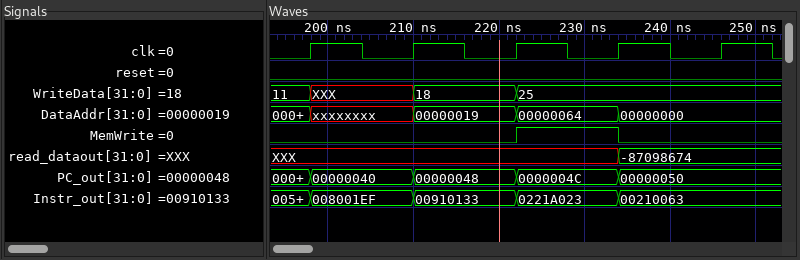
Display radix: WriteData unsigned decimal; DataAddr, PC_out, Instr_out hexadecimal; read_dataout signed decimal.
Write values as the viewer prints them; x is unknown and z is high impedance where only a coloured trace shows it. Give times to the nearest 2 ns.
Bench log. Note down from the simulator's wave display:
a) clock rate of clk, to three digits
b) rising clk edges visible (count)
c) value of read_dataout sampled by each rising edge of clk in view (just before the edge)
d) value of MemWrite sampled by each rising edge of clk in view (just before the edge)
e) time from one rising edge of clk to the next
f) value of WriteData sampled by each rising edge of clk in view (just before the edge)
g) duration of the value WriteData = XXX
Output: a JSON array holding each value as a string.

["83.3 MHz", "5", "XXX, XXX, XXX, XXX, -87098674", "0 0 0 1 0", "12 ns", "11, XXX, 18, 25, 25", "12 ns"]
